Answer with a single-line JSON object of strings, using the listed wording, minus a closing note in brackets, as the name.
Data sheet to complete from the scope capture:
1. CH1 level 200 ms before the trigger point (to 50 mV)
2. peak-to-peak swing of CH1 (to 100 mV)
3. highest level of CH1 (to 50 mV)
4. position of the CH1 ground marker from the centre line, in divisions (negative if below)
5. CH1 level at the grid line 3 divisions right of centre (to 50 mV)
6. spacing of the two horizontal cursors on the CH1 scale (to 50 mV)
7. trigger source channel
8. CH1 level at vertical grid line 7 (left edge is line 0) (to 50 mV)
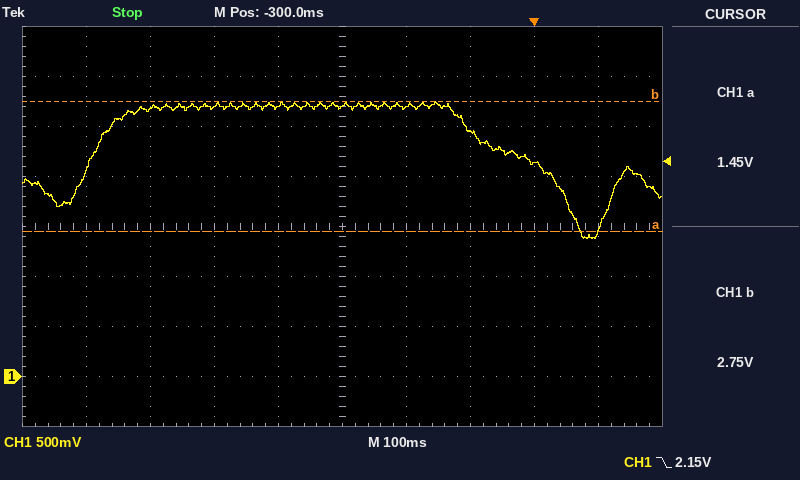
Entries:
{"CH1 level 200 ms before the trigger point": "2.70 V", "peak-to-peak swing of CH1": "1.40 V", "highest level of CH1": "2.75 V", "position of the CH1 ground marker from the centre line, in divisions": "-3.0 div", "CH1 level at the grid line 3 divisions right of centre": "2.15 V", "spacing of the two horizontal cursors on the CH1 scale": "1.30 V", "trigger source channel": "CH1", "CH1 level at vertical grid line 7 (left edge is line 0)": "2.45 V"}
